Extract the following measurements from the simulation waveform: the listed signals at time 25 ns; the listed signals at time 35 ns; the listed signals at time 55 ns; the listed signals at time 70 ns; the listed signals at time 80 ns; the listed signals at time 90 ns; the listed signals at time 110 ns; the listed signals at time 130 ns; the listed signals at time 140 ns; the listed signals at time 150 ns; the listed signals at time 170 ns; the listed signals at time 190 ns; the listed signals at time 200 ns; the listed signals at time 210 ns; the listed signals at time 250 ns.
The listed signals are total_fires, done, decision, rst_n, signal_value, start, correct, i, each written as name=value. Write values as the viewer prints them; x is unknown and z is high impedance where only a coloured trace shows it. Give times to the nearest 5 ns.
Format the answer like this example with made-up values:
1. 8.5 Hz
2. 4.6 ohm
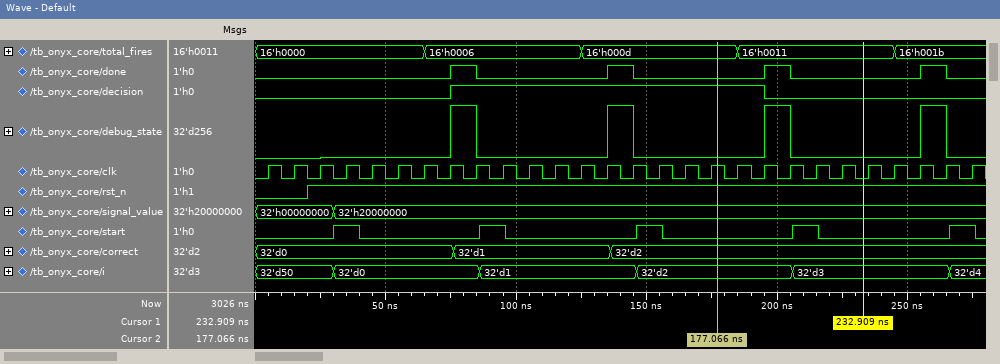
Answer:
1. total_fires=16'h0000, done=0, decision=0, rst_n=1, signal_value=32'h00000000, start=0, correct=32'd0, i=32'd50
2. total_fires=16'h0000, done=0, decision=0, rst_n=1, signal_value=32'h20000000, start=1, correct=32'd0, i=32'd0
3. total_fires=16'h0000, done=0, decision=0, rst_n=1, signal_value=32'h20000000, start=0, correct=32'd0, i=32'd0
4. total_fires=16'h0006, done=0, decision=0, rst_n=1, signal_value=32'h20000000, start=0, correct=32'd0, i=32'd0
5. total_fires=16'h0006, done=1, decision=1, rst_n=1, signal_value=32'h20000000, start=0, correct=32'd1, i=32'd0
6. total_fires=16'h0006, done=0, decision=1, rst_n=1, signal_value=32'h20000000, start=1, correct=32'd1, i=32'd1
7. total_fires=16'h0006, done=0, decision=1, rst_n=1, signal_value=32'h20000000, start=0, correct=32'd1, i=32'd1
8. total_fires=16'h000d, done=0, decision=1, rst_n=1, signal_value=32'h20000000, start=0, correct=32'd1, i=32'd1
9. total_fires=16'h000d, done=1, decision=1, rst_n=1, signal_value=32'h20000000, start=0, correct=32'd2, i=32'd1
10. total_fires=16'h000d, done=0, decision=1, rst_n=1, signal_value=32'h20000000, start=1, correct=32'd2, i=32'd2
11. total_fires=16'h000d, done=0, decision=1, rst_n=1, signal_value=32'h20000000, start=0, correct=32'd2, i=32'd2
12. total_fires=16'h0011, done=0, decision=1, rst_n=1, signal_value=32'h20000000, start=0, correct=32'd2, i=32'd2
13. total_fires=16'h0011, done=1, decision=0, rst_n=1, signal_value=32'h20000000, start=0, correct=32'd2, i=32'd2
14. total_fires=16'h0011, done=0, decision=0, rst_n=1, signal_value=32'h20000000, start=1, correct=32'd2, i=32'd3
15. total_fires=16'h001b, done=0, decision=0, rst_n=1, signal_value=32'h20000000, start=0, correct=32'd2, i=32'd3
